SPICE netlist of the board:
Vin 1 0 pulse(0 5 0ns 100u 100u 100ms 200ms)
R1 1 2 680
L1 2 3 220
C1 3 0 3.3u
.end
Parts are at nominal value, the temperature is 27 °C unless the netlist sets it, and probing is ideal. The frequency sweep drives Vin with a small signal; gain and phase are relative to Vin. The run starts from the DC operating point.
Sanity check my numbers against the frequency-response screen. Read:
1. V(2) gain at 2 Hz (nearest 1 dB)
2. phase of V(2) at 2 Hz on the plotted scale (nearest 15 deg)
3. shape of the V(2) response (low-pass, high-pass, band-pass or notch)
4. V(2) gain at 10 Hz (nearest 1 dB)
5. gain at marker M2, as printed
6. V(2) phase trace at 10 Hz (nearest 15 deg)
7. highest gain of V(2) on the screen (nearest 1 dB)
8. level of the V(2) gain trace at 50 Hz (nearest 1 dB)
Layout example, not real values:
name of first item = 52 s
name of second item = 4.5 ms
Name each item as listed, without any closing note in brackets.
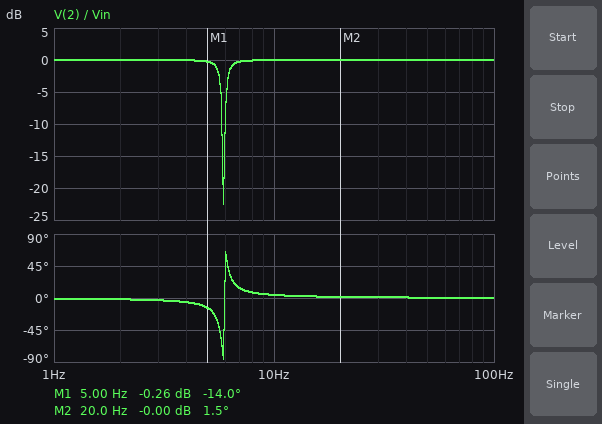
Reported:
V(2) gain at 2 Hz = 0 dB
phase of V(2) at 2 Hz on the plotted scale = 0 deg
shape of the V(2) response = notch
V(2) gain at 10 Hz = 0 dB
gain at marker M2, as printed = -0.00 dB
V(2) phase trace at 10 Hz = 0 deg
highest gain of V(2) on the screen = 0 dB
level of the V(2) gain trace at 50 Hz = 0 dB
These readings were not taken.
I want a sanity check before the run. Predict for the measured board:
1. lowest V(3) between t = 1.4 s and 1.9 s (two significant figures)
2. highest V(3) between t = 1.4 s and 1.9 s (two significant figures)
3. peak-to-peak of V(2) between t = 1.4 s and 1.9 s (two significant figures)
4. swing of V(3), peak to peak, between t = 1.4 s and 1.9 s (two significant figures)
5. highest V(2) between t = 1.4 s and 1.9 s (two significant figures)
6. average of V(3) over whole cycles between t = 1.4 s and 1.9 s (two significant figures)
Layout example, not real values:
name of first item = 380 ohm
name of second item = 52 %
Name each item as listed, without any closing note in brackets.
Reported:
lowest V(3) between t = 1.4 s and 1.9 s = -9.2 V
highest V(3) between t = 1.4 s and 1.9 s = 14 V
peak-to-peak of V(2) between t = 1.4 s and 1.9 s = 6.4 V
swing of V(3), peak to peak, between t = 1.4 s and 1.9 s = 23 V
highest V(2) between t = 1.4 s and 1.9 s = 5.7 V
average of V(3) over whole cycles between t = 1.4 s and 1.9 s = 2.5 V
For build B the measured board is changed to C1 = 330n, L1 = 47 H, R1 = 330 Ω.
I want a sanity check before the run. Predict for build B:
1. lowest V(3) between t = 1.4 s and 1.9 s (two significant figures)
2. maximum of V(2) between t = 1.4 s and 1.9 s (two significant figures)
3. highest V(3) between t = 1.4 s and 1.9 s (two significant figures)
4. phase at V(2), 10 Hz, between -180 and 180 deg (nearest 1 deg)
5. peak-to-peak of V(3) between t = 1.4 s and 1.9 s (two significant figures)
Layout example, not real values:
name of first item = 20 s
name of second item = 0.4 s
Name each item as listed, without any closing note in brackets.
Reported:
lowest V(3) between t = 1.4 s and 1.9 s = -2.9 V
maximum of V(2) between t = 1.4 s and 1.9 s = 5.1 V
highest V(3) between t = 1.4 s and 1.9 s = 7.7 V
phase at V(2), 10 Hz, between -180 and 180 deg = 0 deg
peak-to-peak of V(3) between t = 1.4 s and 1.9 s = 11 V
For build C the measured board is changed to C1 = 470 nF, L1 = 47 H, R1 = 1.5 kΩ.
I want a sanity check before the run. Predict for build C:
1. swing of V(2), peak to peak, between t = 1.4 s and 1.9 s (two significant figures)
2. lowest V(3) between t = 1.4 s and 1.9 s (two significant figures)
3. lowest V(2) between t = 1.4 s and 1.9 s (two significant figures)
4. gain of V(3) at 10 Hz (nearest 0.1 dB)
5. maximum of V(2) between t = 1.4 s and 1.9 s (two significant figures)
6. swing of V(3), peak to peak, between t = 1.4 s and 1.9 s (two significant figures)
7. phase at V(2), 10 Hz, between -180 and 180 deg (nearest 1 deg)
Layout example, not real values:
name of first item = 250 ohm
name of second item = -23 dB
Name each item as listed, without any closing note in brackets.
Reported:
swing of V(2), peak to peak, between t = 1.4 s and 1.9 s = 6.2 V
lowest V(3) between t = 1.4 s and 1.9 s = -4.5 V
lowest V(2) between t = 1.4 s and 1.9 s = -600 mV
gain of V(3) at 10 Hz = 0.8 dB
maximum of V(2) between t = 1.4 s and 1.9 s = 5.6 V
swing of V(3), peak to peak, between t = 1.4 s and 1.9 s = 14 V
phase at V(2), 10 Hz, between -180 and 180 deg = -3 deg
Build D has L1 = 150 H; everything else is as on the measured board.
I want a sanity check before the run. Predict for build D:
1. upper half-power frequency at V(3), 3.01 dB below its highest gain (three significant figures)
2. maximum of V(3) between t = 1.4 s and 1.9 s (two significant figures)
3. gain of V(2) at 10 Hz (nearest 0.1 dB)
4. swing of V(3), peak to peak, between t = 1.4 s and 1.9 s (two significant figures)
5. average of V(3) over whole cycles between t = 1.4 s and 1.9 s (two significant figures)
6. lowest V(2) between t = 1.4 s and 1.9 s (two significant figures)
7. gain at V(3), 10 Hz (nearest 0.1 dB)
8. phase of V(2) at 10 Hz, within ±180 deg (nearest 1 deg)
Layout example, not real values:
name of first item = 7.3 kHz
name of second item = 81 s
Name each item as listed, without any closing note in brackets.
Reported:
upper half-power frequency at V(3), 3.01 dB below its highest gain = 7.49 Hz
maximum of V(3) between t = 1.4 s and 1.9 s = 9.0 V
gain of V(2) at 10 Hz = -0.1 dB
swing of V(3), peak to peak, between t = 1.4 s and 1.9 s = 13 V
average of V(3) over whole cycles between t = 1.4 s and 1.9 s = 2.5 V
lowest V(2) between t = 1.4 s and 1.9 s = -370 mV
gain at V(3), 10 Hz = 0.3 dB
phase of V(2) at 10 Hz, within ±180 deg = 8 deg
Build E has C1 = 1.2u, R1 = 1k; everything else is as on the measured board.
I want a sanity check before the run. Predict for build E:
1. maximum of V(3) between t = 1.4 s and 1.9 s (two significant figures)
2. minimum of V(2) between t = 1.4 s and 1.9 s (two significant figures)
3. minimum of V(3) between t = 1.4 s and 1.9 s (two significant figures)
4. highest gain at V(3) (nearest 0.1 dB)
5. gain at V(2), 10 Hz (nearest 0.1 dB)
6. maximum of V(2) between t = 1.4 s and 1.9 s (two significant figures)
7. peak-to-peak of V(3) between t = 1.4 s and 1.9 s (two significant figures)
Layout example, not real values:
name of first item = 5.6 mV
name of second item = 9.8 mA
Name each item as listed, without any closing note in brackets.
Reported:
maximum of V(3) between t = 1.4 s and 1.9 s = 7.5 V
minimum of V(2) between t = 1.4 s and 1.9 s = -170 mV
minimum of V(3) between t = 1.4 s and 1.9 s = -2.5 V
highest gain at V(3) = 22.6 dB
gain at V(2), 10 Hz = -6.2 dB
maximum of V(2) between t = 1.4 s and 1.9 s = 5.2 V
peak-to-peak of V(3) between t = 1.4 s and 1.9 s = 10 V
